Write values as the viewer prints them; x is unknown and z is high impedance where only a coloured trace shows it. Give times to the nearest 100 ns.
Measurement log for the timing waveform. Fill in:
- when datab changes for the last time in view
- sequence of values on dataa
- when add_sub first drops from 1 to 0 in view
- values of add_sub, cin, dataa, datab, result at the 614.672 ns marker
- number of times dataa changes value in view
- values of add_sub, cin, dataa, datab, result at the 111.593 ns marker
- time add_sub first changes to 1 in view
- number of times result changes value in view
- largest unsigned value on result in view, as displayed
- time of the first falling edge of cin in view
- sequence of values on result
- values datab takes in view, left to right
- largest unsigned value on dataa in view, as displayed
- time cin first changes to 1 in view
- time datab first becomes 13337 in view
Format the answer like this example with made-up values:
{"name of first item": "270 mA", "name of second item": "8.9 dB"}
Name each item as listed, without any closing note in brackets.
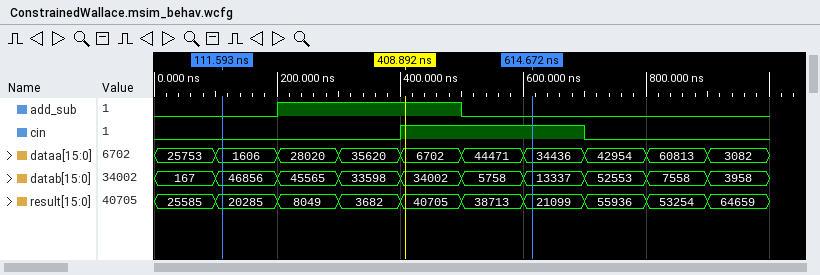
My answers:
{"when datab changes for the last time in view": "900 ns", "sequence of values on dataa": "25753, 1606, 28020, 35620, 6702, 44471, 34436, 42954, 60813, 3082", "when add_sub first drops from 1 to 0 in view": "500 ns", "values of add_sub, cin, dataa, datab, result at the 614.672 ns marker": "add_sub=0, cin=1, dataa=34436, datab=13337, result=21099", "number of times dataa changes value in view": "9", "values of add_sub, cin, dataa, datab, result at the 111.593 ns marker": "add_sub=0, cin=0, dataa=1606, datab=46856, result=20285", "time add_sub first changes to 1 in view": "200 ns", "number of times result changes value in view": "9", "largest unsigned value on result in view, as displayed": "64659", "time of the first falling edge of cin in view": "700 ns", "sequence of values on result": "25585, 20285, 8049, 3682, 40705, 38713, 21099, 55936, 53254, 64659", "values datab takes in view, left to right": "167, 46856, 45565, 33598, 34002, 5758, 13337, 52553, 7558, 3958", "largest unsigned value on dataa in view, as displayed": "60813", "time cin first changes to 1 in view": "400 ns", "time datab first becomes 13337 in view": "600 ns"}
